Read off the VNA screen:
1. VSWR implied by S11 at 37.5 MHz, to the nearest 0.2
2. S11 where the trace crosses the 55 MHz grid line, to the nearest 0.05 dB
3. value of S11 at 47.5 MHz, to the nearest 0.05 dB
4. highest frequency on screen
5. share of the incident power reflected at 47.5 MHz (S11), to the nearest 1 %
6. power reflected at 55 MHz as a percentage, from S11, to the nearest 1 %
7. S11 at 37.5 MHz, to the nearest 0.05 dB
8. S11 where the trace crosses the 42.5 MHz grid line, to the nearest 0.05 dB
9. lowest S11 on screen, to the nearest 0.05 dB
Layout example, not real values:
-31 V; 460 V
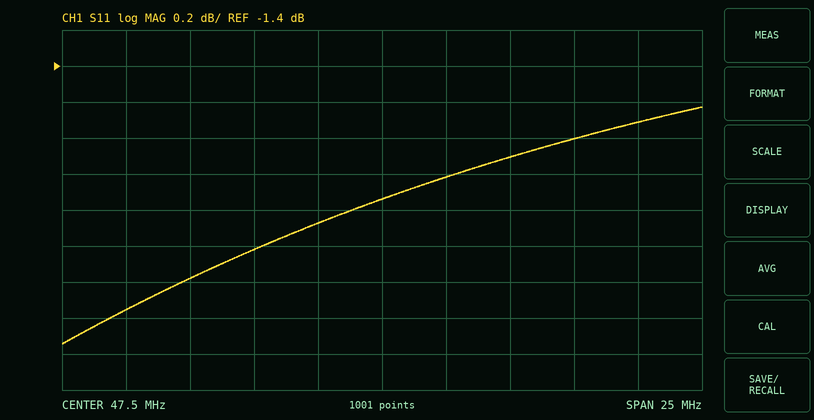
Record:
6.4; -1.80 dB; -2.15 dB; 60 MHz; 61 %; 66 %; -2.75 dB; -2.40 dB; -2.95 dB
